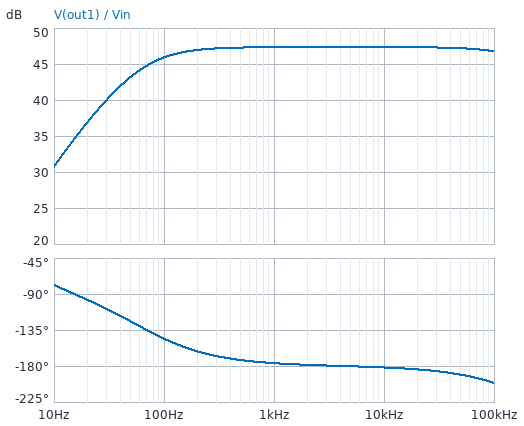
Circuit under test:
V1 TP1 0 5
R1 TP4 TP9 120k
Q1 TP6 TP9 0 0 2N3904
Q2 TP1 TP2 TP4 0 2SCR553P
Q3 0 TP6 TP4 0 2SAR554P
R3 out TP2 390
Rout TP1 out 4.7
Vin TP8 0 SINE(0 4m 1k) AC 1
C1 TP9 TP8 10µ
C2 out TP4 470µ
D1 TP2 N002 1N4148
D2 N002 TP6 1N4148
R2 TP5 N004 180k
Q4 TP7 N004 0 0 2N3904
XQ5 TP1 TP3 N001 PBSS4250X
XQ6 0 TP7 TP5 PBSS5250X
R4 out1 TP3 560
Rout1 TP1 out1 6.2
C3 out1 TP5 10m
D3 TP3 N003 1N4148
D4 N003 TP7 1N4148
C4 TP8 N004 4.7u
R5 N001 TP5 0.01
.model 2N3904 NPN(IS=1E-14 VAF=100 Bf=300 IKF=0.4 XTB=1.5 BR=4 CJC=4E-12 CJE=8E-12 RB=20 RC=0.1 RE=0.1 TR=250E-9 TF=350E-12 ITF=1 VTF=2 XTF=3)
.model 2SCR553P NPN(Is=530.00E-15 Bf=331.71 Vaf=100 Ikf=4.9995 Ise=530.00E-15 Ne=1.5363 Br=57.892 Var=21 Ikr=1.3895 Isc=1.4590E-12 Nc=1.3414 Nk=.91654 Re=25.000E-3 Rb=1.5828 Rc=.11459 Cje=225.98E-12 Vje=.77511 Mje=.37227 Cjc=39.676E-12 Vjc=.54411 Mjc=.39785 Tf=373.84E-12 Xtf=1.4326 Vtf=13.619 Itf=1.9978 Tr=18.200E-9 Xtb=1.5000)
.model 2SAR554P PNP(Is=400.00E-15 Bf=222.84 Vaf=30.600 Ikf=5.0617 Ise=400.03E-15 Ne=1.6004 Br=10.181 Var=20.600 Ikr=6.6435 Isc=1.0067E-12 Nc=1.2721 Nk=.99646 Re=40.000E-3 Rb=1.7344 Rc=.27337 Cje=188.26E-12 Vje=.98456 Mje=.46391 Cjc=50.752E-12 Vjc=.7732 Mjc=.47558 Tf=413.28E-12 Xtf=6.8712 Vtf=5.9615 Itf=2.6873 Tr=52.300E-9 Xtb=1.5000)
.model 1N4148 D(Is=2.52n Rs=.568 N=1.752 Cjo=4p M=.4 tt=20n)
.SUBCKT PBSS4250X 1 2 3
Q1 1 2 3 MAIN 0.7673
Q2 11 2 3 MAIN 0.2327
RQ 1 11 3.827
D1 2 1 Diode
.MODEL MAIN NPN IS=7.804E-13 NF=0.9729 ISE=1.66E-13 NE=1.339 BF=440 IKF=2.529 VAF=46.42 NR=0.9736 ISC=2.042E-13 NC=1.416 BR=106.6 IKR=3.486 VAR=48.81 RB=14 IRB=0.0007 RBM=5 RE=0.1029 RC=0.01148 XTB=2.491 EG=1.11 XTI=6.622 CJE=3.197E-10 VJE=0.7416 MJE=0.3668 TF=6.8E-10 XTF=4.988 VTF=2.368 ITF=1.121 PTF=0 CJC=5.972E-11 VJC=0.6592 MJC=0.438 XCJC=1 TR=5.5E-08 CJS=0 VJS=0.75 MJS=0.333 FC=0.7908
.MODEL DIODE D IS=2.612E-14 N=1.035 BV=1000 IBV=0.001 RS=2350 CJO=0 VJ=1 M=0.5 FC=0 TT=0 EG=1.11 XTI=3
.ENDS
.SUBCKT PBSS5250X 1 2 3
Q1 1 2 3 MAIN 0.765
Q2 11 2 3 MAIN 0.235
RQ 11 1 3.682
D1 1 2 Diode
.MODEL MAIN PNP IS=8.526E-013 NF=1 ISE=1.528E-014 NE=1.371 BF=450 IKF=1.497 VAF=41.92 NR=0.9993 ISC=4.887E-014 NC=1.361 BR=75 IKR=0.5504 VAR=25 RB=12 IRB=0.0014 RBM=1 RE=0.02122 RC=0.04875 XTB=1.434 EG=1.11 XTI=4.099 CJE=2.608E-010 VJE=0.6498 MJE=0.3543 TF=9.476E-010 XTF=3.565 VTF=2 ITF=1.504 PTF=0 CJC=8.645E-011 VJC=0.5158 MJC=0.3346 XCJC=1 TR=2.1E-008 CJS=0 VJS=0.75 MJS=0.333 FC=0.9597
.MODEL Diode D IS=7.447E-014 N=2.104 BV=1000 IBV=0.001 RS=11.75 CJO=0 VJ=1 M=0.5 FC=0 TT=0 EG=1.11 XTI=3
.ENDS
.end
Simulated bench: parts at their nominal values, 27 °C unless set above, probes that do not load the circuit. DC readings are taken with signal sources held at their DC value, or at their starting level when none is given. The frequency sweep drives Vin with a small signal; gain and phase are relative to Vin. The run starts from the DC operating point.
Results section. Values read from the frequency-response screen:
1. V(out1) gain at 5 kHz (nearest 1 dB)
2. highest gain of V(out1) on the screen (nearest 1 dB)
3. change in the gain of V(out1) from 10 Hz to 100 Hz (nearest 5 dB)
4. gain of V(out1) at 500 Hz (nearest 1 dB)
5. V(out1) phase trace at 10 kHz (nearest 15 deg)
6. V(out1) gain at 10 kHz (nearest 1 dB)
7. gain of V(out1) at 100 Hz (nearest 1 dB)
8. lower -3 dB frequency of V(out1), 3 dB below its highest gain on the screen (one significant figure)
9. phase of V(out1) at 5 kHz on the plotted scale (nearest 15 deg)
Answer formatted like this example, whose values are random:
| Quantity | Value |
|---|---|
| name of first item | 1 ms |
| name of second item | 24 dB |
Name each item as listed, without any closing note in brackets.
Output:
| Quantity | Value |
|---|---|
| V(out1) gain at 5 kHz | 47 dB |
| highest gain of V(out1) on the screen | 47 dB |
| change in the gain of V(out1) from 10 Hz to 100 Hz | 15 dB |
| gain of V(out1) at 500 Hz | 47 dB |
| V(out1) phase trace at 10 kHz | -180 deg |
| V(out1) gain at 10 kHz | 47 dB |
| gain of V(out1) at 100 Hz | 46 dB |
| lower -3 dB frequency of V(out1), 3 dB below its highest gain on the screen | 60 Hz |
| phase of V(out1) at 5 kHz on the plotted scale | -180 deg |
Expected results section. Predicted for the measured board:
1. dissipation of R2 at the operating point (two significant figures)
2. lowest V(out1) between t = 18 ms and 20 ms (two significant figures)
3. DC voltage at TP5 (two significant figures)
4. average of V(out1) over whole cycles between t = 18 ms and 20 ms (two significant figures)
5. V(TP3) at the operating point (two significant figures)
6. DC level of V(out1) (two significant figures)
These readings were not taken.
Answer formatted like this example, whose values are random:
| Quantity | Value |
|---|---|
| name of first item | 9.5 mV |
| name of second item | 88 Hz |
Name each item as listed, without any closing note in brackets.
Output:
| Quantity | Value |
|---|---|
| dissipation of R2 at the operating point | 20 µW |
| lowest V(out1) between t = 18 ms and 20 ms | 4.0 V |
| DC voltage at TP5 | 2.6 V |
| average of V(out1) over whole cycles between t = 18 ms and 20 ms | 5.0 V |
| V(TP3) at the operating point | 3.2 V |
| DC level of V(out1) | 5.0 V |
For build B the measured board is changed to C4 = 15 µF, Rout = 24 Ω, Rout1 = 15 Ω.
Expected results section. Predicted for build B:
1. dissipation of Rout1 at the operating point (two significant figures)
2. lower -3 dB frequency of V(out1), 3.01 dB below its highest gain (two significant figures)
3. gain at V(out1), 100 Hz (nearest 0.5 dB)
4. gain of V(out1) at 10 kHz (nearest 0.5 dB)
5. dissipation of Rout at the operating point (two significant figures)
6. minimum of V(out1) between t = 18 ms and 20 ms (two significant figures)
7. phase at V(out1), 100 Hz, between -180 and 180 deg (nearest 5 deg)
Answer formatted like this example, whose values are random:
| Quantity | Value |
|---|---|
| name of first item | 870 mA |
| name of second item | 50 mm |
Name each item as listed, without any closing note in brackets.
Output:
| Quantity | Value |
|---|---|
| dissipation of Rout1 at the operating point | 150 µW |
| lower -3 dB frequency of V(out1), 3.01 dB below its highest gain | 41 Hz |
| gain at V(out1), 100 Hz | 53.5 dB |
| gain of V(out1) at 10 kHz | 54.0 dB |
| dissipation of Rout at the operating point | 480 µW |
| minimum of V(out1) between t = 18 ms and 20 ms | 3.2 V |
| phase at V(out1), 100 Hz, between -180 and 180 deg | -155 deg |
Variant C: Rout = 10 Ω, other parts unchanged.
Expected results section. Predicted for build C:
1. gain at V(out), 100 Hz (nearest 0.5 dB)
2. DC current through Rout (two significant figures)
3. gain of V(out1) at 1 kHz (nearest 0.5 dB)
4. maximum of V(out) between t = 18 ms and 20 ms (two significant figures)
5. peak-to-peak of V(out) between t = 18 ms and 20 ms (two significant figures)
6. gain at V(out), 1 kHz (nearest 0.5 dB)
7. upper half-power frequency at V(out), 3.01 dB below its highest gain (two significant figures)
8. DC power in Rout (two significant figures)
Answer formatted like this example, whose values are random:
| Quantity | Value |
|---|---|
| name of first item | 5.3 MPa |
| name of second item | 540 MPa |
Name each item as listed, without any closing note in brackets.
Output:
| Quantity | Value |
|---|---|
| gain at V(out), 100 Hz | 43.0 dB |
| DC current through Rout | 4.5 mA |
| gain of V(out1) at 1 kHz | 47.5 dB |
| maximum of V(out) between t = 18 ms and 20 ms | 6.2 V |
| peak-to-peak of V(out) between t = 18 ms and 20 ms | 2.5 V |
| gain at V(out), 1 kHz | 50.0 dB |
| upper half-power frequency at V(out), 3.01 dB below its highest gain | 660 kHz |
| DC power in Rout | 210 µW |
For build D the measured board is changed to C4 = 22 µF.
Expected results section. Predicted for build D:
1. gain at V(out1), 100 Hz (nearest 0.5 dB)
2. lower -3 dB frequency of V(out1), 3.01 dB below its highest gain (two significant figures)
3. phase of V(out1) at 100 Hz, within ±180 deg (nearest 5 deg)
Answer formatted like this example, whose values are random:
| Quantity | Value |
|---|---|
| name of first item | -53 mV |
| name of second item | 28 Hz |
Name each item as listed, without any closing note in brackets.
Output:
| Quantity | Value |
|---|---|
| gain at V(out1), 100 Hz | 47.0 dB |
| lower -3 dB frequency of V(out1), 3.01 dB below its highest gain | 19 Hz |
| phase of V(out1) at 100 Hz, within ±180 deg | -170 deg |
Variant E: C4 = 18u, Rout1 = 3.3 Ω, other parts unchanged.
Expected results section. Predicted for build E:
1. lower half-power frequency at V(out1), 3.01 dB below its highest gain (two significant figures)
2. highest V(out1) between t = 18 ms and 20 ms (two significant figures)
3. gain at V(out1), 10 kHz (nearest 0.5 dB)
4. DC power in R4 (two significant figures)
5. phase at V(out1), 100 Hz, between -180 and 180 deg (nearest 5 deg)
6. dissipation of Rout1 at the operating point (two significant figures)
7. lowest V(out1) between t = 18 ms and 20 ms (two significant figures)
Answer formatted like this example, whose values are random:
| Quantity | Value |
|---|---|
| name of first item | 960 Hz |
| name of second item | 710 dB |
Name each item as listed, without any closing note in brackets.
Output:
| Quantity | Value |
|---|---|
| lower half-power frequency at V(out1), 3.01 dB below its highest gain | 16 Hz |
| highest V(out1) between t = 18 ms and 20 ms | 5.5 V |
| gain at V(out1), 10 kHz | 42.0 dB |
| DC power in R4 | 5.7 mW |
| phase at V(out1), 100 Hz, between -180 and 180 deg | -170 deg |
| dissipation of Rout1 at the operating point | 33 µW |
| lowest V(out1) between t = 18 ms and 20 ms | 4.5 V |
